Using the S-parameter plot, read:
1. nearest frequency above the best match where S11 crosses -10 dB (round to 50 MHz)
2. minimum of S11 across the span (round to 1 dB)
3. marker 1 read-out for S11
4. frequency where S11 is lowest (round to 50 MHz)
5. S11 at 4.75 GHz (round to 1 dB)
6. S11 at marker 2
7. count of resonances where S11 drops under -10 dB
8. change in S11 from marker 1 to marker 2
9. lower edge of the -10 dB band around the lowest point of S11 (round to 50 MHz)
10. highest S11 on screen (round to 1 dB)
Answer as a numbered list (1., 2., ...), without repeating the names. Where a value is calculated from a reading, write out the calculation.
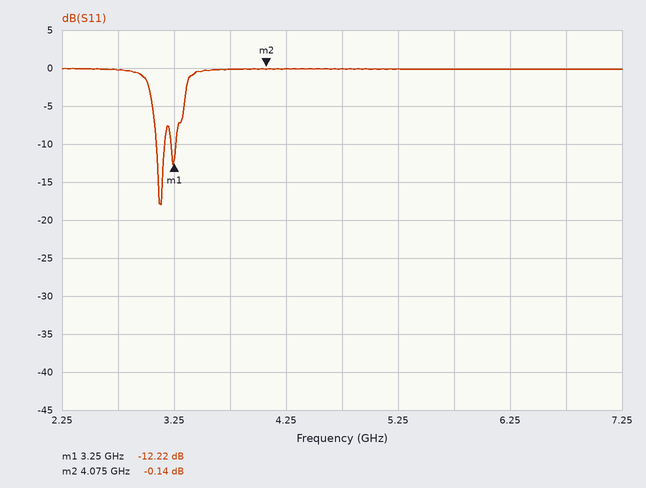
1. 3.15 GHz
2. -18 dB
3. -12.22 dB
4. 3.15 GHz
5. 0 dB
6. -0.14 dB
7. 2
8. -0.14 − (-12.22) = 12.08 dB
9. 3.10 GHz
10. 0 dB
